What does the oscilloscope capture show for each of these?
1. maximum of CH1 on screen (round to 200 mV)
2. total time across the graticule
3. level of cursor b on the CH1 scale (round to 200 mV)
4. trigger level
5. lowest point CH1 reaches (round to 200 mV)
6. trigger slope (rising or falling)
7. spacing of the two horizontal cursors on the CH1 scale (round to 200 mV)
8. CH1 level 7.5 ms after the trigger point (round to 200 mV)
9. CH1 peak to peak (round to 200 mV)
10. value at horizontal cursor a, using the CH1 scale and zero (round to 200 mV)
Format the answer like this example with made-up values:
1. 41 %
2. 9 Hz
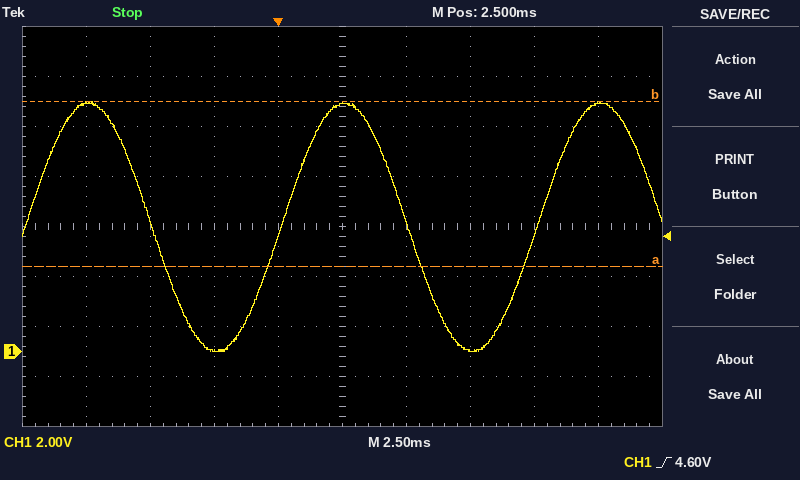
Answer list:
1. 10.0 V
2. 25 ms
3. 10.0 V
4. 4.60 V
5. 0.0 V
6. rising
7. 6.6 V
8. 0.0 V
9. 10.0 V
10. 3.4 V
